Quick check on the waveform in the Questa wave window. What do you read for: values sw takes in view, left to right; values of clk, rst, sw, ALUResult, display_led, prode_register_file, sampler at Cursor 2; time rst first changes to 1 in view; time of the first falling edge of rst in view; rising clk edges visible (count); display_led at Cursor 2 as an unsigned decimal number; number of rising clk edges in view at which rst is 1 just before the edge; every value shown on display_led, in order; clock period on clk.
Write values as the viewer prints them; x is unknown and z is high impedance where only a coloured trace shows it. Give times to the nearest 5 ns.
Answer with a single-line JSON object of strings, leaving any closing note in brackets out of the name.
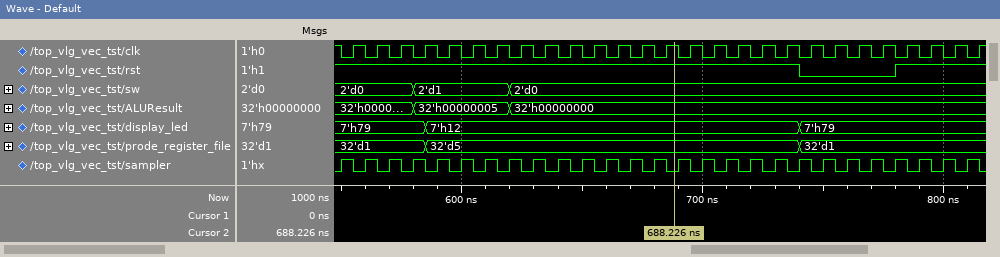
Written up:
{"values sw takes in view, left to right": "2'd0, 2'd1, 2'd0", "values of clk, rst, sw, ALUResult, display_led, prode_register_file, sampler at Cursor 2": "clk=1, rst=1, sw=2'd0, ALUResult=32'h00000000, display_led=7'h12, prode_register_file=32'd5, sampler=0", "time rst first changes to 1 in view": "780 ns", "time of the first falling edge of rst in view": "740 ns", "rising clk edges visible": "27", "display_led at Cursor 2 as an unsigned decimal number": "18", "number of rising clk edges in view at which rst is 1 just before the edge": "23", "every value shown on display_led, in order": "7'h79, 7'h12, 7'h79", "clock period on clk": "10 ns"}
